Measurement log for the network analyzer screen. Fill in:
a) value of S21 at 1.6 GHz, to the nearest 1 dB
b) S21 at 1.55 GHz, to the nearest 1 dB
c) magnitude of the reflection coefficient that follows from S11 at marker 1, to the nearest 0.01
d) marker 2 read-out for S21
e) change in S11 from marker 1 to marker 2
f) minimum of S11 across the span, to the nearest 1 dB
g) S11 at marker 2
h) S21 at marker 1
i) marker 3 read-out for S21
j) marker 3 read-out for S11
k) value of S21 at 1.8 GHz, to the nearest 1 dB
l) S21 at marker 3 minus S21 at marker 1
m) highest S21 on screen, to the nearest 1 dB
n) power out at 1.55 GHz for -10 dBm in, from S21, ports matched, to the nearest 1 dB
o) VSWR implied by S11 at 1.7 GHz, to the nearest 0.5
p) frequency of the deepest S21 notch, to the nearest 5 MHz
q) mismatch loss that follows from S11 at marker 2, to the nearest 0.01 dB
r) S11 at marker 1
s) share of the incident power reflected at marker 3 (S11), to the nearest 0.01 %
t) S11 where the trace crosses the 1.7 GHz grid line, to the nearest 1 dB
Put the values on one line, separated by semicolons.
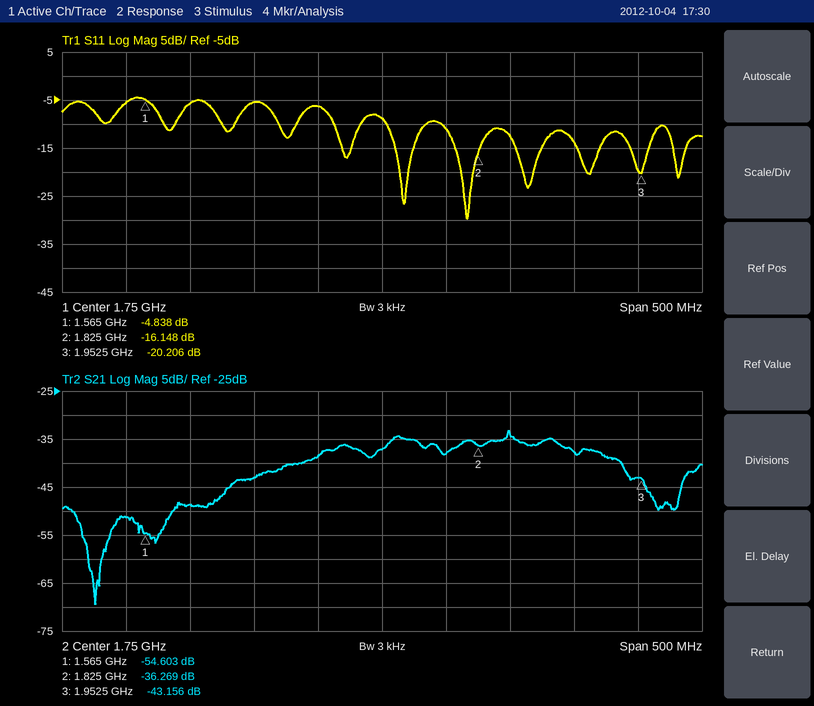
-49 dB; -51 dB; 0.57; -36.269 dB; -11.310 dB; -30 dB; -16.148 dB; -54.603 dB; -43.156 dB; -20.206 dB; -38 dB; 11.447 dB; -33 dB; -61 dBm; 3.0; 1.525 GHz; 0.11 dB; -4.838 dB; 0.95 %; -6 dB
